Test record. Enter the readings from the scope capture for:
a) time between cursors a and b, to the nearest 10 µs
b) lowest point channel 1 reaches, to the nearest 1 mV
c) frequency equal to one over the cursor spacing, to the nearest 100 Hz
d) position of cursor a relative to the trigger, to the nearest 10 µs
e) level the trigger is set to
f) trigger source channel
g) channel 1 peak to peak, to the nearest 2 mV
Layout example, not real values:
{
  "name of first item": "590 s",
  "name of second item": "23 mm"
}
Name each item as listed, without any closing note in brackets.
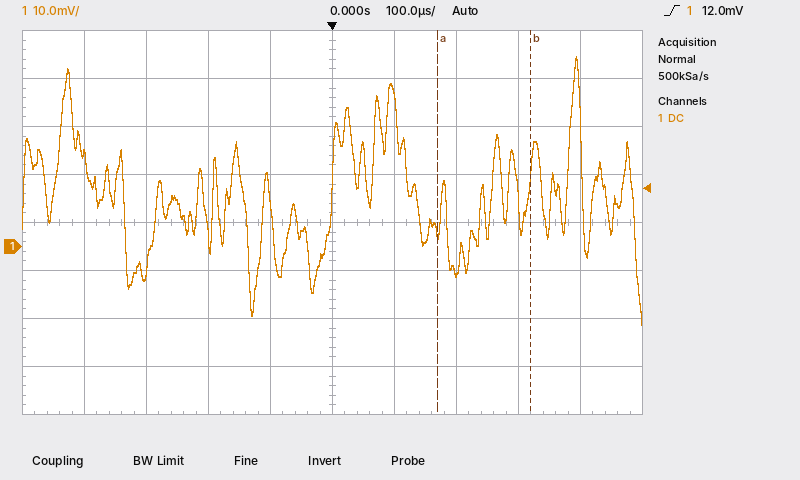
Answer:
{
  "time between cursors a and b, to the nearest 10 µs": "150 µs",
  "lowest point channel 1 reaches, to the nearest 1 mV": "-16 mV",
  "frequency equal to one over the cursor spacing, to the nearest 100 Hz": "6.7 kHz",
  "position of cursor a relative to the trigger, to the nearest 10 µs": "+170 µs",
  "level the trigger is set to": "12.0 mV",
  "trigger source channel": "channel 1",
  "channel 1 peak to peak, to the nearest 2 mV": "56 mV"
}
